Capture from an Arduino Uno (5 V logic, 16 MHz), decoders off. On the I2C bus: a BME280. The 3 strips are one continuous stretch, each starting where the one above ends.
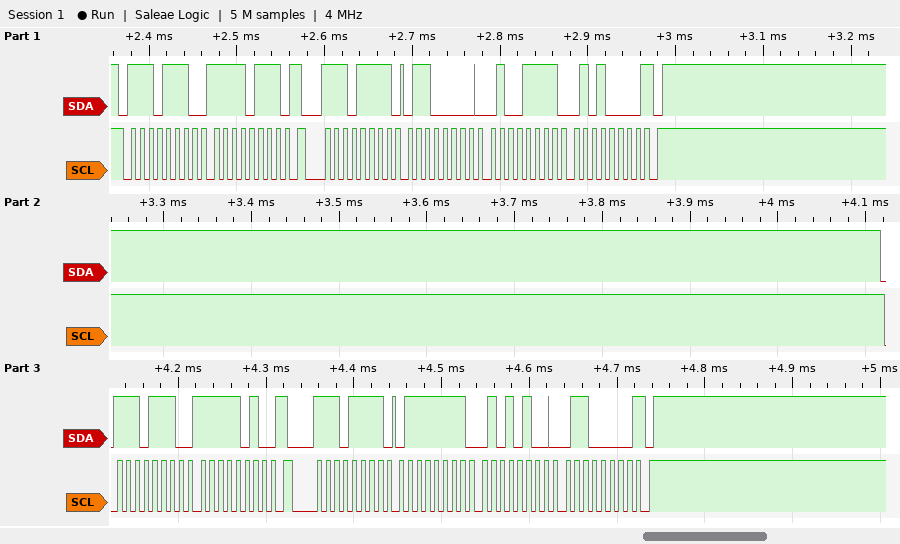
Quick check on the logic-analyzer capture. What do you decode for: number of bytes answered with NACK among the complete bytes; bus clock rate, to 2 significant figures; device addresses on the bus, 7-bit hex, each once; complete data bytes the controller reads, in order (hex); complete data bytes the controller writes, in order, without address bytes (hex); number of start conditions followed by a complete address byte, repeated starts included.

2
100 kHz
0x77
60 4F 50 7F 54 60
F7 FA
4
